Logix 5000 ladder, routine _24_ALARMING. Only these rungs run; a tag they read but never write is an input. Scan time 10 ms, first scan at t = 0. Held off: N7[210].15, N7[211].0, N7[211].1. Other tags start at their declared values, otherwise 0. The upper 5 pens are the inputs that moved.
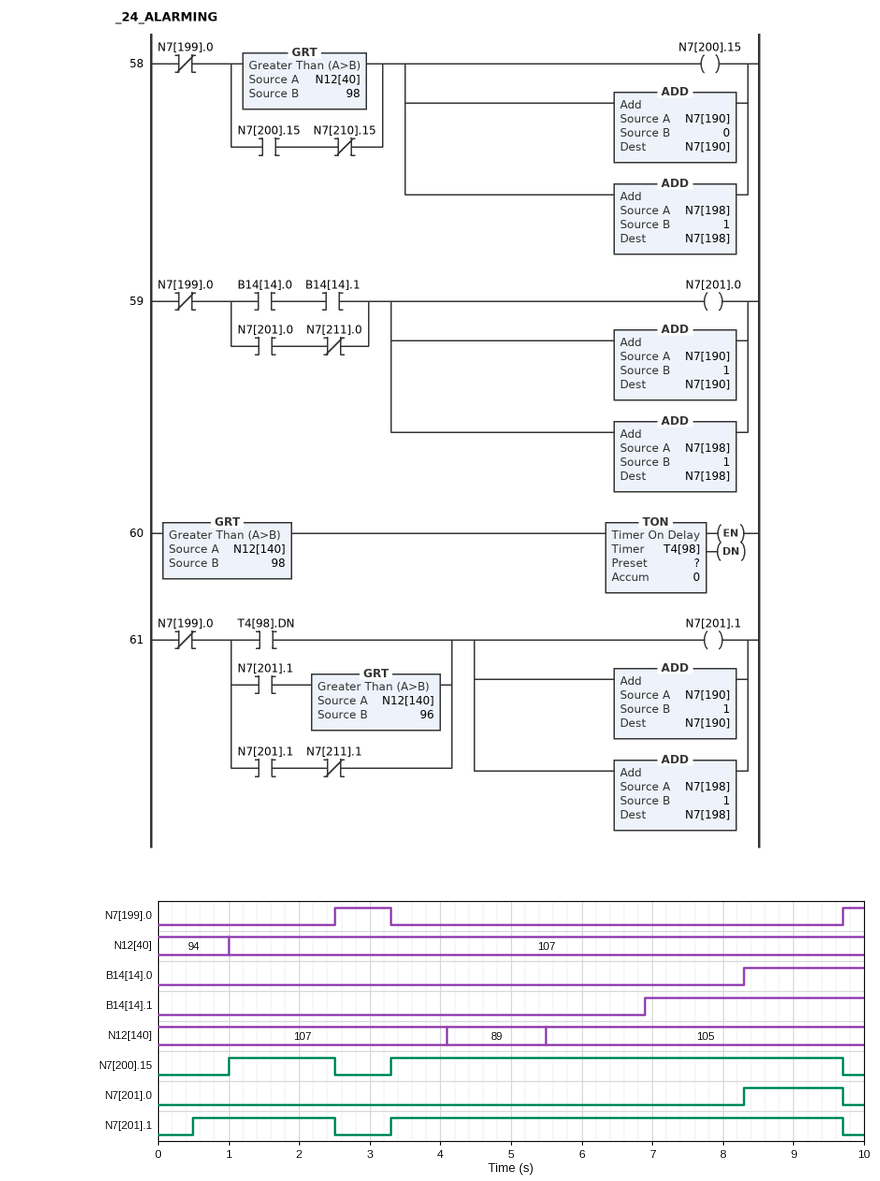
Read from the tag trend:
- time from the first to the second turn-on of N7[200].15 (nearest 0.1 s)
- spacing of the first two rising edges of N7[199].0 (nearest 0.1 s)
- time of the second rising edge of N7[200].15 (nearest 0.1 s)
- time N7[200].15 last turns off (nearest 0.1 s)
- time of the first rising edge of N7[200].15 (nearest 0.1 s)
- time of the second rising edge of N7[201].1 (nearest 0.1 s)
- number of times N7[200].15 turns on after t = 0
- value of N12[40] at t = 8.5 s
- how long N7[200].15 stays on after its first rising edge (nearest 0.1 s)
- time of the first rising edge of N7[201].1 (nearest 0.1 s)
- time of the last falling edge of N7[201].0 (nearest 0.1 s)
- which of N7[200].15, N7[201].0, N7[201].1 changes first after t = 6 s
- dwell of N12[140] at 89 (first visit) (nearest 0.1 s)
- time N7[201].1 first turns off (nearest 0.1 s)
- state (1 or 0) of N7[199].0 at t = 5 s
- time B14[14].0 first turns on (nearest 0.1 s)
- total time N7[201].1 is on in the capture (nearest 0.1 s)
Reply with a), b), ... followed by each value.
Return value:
a) 2.3 s
b) 7.2 s
c) 3.3 s
d) 9.7 s
e) 1.0 s
f) 3.3 s
g) 2
h) 107
i) 1.5 s
j) 0.5 s
k) 9.7 s
l) N7[201].0
m) 1.4 s
n) 2.5 s
o) 0
p) 8.3 s
q) 8.4 s
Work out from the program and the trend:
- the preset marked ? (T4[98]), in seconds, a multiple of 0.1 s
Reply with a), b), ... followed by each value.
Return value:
a) 0.5 s
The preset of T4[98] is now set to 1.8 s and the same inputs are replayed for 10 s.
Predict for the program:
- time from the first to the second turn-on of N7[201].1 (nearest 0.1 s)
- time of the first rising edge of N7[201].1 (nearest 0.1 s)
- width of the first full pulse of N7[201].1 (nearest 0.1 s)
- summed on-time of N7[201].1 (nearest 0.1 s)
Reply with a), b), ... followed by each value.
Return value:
a) 1.5 s
b) 1.8 s
c) 0.7 s
d) 7.1 s
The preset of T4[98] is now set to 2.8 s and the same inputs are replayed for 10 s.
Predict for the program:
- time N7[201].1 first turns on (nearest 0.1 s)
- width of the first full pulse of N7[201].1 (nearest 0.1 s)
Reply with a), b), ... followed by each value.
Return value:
a) 3.3 s
b) 6.4 s
